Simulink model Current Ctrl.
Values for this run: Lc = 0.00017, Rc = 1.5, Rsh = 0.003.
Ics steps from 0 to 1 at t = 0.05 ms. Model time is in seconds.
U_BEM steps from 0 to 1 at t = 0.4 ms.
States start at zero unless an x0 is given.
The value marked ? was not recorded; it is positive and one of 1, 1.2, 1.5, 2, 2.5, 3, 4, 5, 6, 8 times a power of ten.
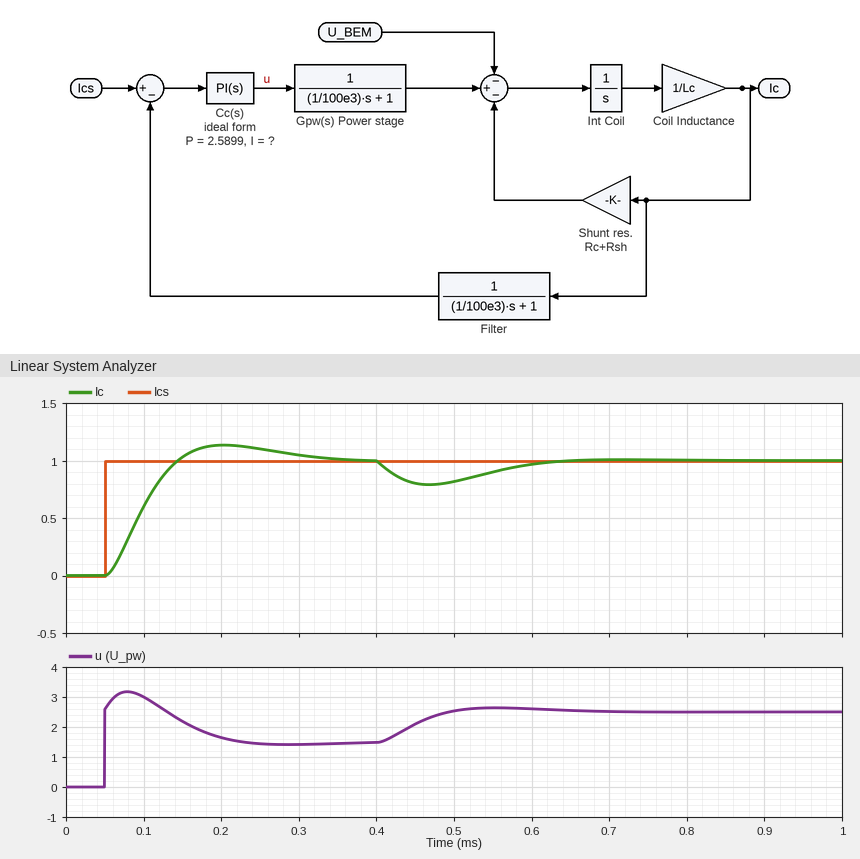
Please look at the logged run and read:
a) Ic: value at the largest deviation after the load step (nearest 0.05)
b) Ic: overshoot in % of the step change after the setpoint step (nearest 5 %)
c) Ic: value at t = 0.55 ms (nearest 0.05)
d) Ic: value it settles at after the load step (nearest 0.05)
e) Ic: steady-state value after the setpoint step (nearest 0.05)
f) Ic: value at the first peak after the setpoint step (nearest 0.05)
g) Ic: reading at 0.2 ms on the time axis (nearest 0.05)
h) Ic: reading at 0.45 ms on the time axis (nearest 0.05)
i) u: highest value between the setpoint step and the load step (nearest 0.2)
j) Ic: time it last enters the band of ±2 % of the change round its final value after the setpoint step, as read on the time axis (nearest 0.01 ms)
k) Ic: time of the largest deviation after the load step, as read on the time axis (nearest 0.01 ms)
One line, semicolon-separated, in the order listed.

0.80; 15 %; 0.90; 1.00; 1.00; 1.15; 1.15; 0.80; 3.2; 0.34 ms; 0.47 ms
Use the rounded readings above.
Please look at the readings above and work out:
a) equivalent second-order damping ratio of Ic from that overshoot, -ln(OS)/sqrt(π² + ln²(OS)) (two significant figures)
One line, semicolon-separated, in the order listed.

0.52
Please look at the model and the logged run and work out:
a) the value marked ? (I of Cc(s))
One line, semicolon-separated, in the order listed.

15000
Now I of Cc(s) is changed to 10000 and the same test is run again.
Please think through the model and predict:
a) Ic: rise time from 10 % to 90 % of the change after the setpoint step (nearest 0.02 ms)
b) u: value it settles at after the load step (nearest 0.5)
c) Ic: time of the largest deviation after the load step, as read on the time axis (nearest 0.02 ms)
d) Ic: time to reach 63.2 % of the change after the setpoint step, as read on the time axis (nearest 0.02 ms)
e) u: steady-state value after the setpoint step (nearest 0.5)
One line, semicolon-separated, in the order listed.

0.08 ms; 2.5; 0.48 ms; 0.10 ms; 1.5
